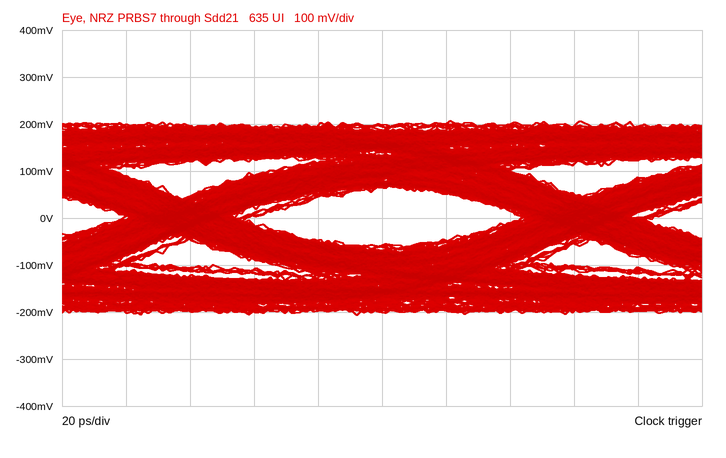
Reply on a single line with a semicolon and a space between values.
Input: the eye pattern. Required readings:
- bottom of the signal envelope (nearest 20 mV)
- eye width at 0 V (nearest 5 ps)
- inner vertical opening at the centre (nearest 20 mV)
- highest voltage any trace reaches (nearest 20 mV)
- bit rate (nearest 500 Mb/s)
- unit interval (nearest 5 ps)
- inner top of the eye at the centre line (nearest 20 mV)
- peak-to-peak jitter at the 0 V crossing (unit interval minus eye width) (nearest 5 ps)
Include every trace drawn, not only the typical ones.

-200 mV; 85 ps; 120 mV; 200 mV; 8.0 Gb/s; 125 ps; 60 mV; 40 ps
